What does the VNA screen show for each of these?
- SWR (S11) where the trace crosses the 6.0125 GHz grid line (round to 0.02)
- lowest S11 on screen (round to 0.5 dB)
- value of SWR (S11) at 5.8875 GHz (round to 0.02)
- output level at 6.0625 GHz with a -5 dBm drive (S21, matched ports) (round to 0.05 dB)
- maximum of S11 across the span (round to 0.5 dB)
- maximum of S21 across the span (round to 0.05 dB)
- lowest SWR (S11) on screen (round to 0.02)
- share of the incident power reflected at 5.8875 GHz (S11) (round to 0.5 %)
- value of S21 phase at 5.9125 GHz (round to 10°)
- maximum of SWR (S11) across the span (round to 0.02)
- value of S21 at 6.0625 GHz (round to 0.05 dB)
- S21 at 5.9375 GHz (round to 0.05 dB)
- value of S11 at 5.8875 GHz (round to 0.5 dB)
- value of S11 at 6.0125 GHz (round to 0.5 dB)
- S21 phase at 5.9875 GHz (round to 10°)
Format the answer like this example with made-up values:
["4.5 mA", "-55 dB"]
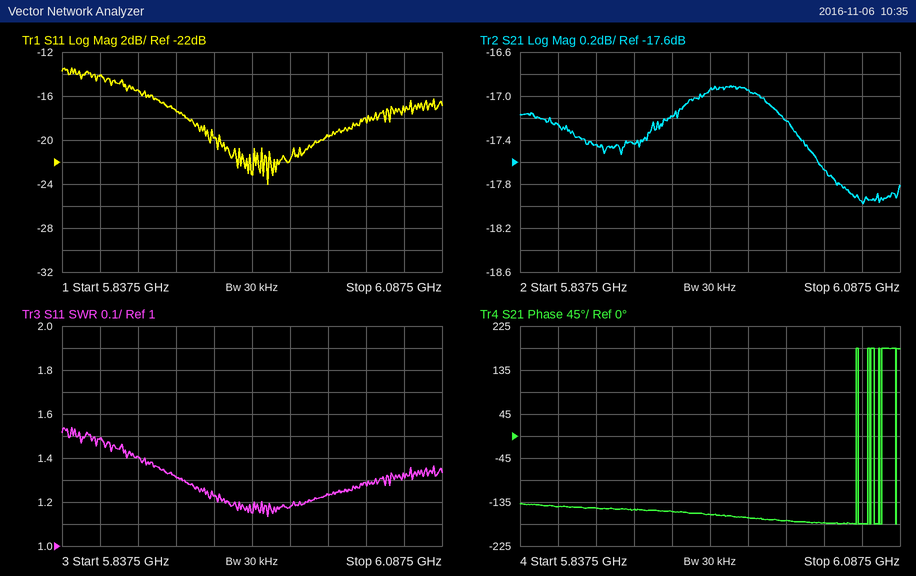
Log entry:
["1.24", "-24.0 dB", "1.40", "-22.95 dBm", "-13.5 dB", "-16.90 dB", "1.14", "3.0 %", "-150°", "1.54", "-17.95 dB", "-17.20 dB", "-15.5 dB", "-19.5 dB", "-170°"]
